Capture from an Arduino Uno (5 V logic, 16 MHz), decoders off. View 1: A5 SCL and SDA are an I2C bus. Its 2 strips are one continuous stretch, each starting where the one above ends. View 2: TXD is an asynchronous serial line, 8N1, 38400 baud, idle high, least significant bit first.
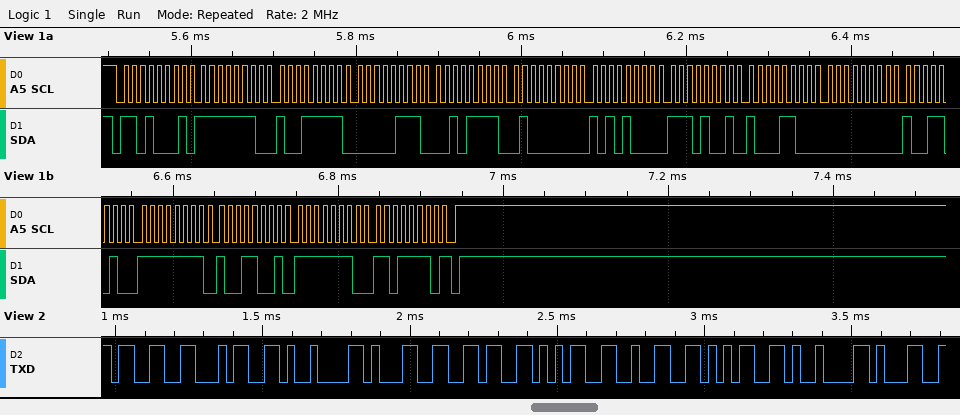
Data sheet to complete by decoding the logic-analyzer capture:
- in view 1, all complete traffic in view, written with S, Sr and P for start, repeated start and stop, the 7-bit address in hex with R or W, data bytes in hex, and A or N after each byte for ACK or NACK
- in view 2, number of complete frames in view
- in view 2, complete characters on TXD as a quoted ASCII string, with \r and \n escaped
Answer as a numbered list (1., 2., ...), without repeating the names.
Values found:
1. S 68R A FE A 9F A 07 A 2F A 40 A A8 A E9 A 8C A 00 A 9A A FF A 99 A FE A DE N P
2. 10
3. "34\t16525\t1"
